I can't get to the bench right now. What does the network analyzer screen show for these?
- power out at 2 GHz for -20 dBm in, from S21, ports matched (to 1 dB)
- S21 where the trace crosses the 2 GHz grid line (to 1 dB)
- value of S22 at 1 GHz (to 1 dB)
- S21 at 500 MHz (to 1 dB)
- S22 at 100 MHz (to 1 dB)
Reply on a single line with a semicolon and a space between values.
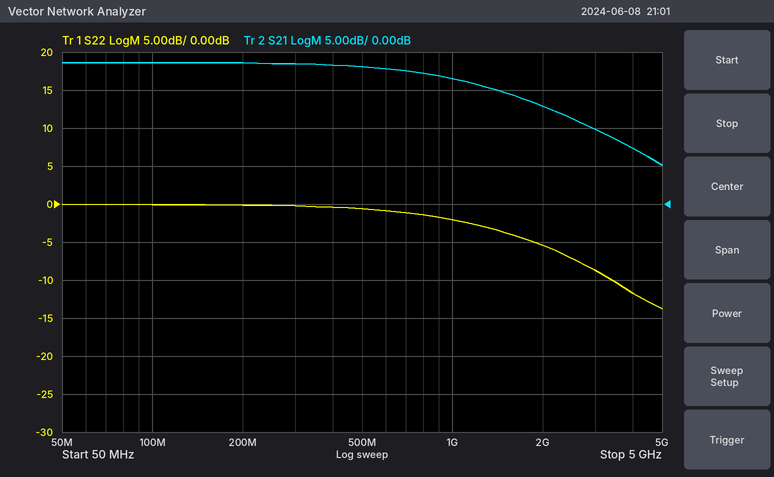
-7 dBm; 13 dB; -2 dB; 18 dB; 0 dB
